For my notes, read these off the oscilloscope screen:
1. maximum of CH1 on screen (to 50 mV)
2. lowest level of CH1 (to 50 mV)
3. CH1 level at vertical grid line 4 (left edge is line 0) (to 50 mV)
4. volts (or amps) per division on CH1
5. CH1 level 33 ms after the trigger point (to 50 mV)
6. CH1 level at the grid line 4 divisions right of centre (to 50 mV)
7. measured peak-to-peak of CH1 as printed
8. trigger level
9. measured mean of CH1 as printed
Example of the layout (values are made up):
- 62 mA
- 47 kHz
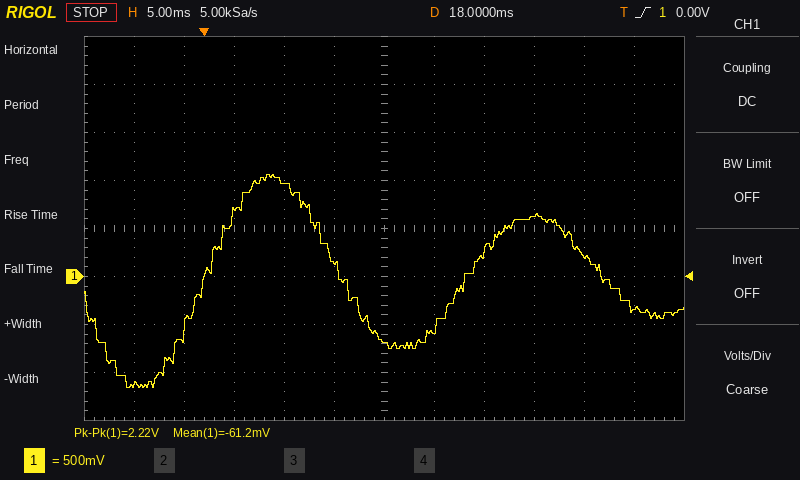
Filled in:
- 1.05 V
- -1.15 V
- 950 mV
- 500 mV
- 650 mV
- 200 mV
- 2.22 V
- 0.00 V
- -61.2 mV
